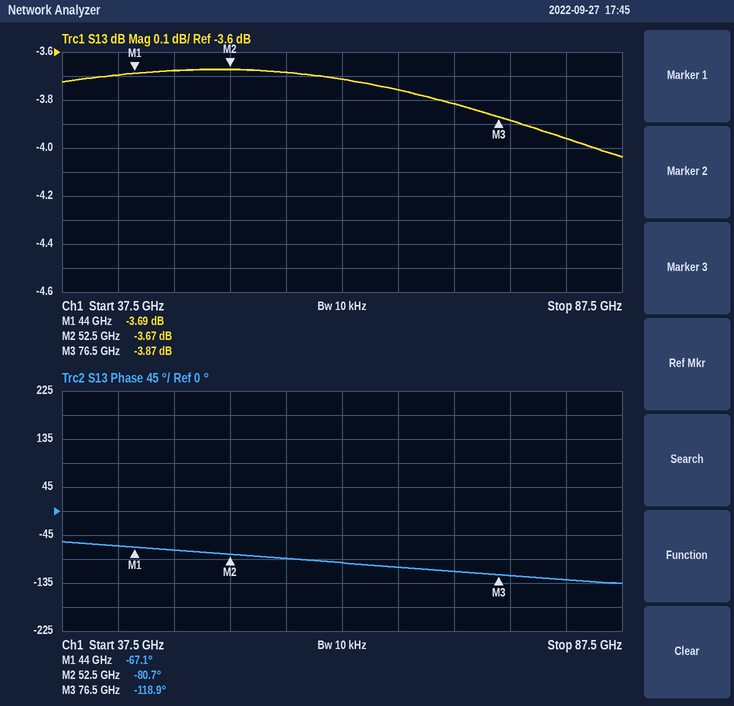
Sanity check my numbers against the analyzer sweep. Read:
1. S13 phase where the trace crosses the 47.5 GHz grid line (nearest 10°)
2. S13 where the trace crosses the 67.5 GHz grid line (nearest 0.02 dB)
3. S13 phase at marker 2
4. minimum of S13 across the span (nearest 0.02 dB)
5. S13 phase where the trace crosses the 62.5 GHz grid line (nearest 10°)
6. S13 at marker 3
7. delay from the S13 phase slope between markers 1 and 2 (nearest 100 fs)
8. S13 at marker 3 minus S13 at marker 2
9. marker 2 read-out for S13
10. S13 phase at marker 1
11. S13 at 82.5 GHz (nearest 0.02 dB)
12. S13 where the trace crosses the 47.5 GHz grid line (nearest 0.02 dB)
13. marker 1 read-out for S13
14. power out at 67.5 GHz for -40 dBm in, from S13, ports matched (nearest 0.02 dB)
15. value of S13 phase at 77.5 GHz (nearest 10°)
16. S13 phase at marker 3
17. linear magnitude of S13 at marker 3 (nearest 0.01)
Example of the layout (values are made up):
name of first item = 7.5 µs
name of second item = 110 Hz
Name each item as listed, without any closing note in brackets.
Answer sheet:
S13 phase where the trace crosses the 47.5 GHz grid line = -70°
S13 where the trace crosses the 67.5 GHz grid line = -3.76 dB
S13 phase at marker 2 = -80.7°
minimum of S13 across the span = -4.04 dB
S13 phase where the trace crosses the 62.5 GHz grid line = -100°
S13 at marker 3 = -3.87 dB
delay from the S13 phase slope between markers 1 and 2 = 4.4 ps
S13 at marker 3 minus S13 at marker 2 = -0.20 dB
marker 2 read-out for S13 = -3.67 dB
S13 phase at marker 1 = -67.1°
S13 at 82.5 GHz = -3.96 dB
S13 where the trace crosses the 47.5 GHz grid line = -3.68 dB
marker 1 read-out for S13 = -3.69 dB
power out at 67.5 GHz for -40 dBm in, from S13, ports matched = -43.76 dBm
value of S13 phase at 77.5 GHz = -120°
S13 phase at marker 3 = -118.9°
linear magnitude of S13 at marker 3 = 0.64
